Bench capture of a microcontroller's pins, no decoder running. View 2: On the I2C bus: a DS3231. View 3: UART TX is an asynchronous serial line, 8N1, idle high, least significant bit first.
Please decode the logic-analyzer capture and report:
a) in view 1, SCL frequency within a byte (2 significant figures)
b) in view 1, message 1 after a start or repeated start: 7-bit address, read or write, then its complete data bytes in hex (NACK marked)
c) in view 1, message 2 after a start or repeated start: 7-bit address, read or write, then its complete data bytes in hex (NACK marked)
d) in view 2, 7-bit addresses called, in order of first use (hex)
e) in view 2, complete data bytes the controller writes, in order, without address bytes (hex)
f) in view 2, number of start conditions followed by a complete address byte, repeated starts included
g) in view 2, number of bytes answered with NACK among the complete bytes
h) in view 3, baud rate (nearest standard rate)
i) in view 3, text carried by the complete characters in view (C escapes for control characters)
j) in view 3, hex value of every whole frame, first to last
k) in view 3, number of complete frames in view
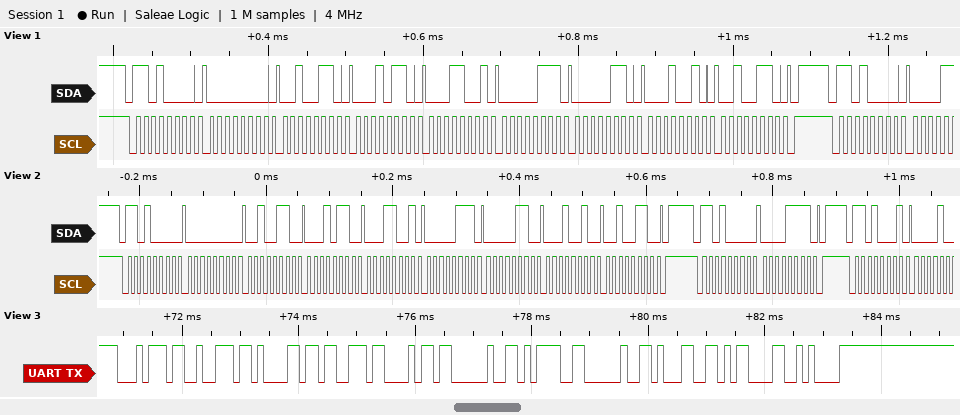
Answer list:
100 kHz
0x68 write: 00 26 16 19 07 06 12 26
0x68 write
0x68
00 26 16 19 07 06 12 26 0F
3
0
9600 baud
"trash = 1\r\n"
74 72 61 73 68 20 3D 20 31 0D 0A
11
